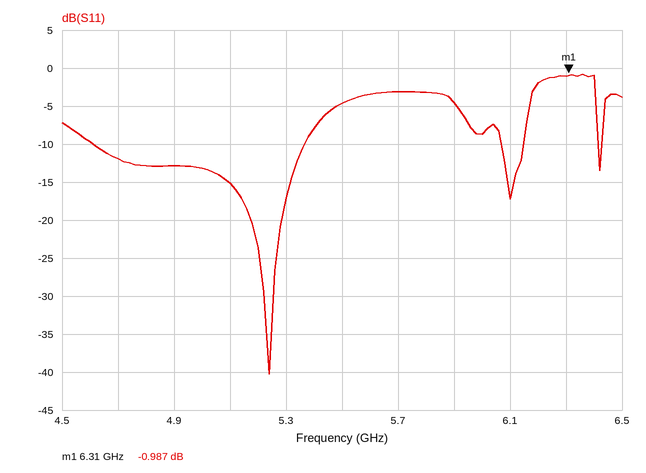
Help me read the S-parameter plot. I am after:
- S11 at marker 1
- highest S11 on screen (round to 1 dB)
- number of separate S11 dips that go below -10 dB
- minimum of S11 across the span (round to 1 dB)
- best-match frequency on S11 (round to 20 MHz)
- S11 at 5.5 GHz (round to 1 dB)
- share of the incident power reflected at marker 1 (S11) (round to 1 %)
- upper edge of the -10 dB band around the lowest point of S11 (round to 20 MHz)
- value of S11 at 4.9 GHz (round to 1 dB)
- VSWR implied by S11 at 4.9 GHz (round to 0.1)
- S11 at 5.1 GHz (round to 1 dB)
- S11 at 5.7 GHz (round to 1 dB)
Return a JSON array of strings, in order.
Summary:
["-0.987 dB", "-1 dB", "3", "-40 dB", "5.24 GHz", "-5 dB", "80 %", "5.36 GHz", "-13 dB", "1.6", "-15 dB", "-3 dB"]
